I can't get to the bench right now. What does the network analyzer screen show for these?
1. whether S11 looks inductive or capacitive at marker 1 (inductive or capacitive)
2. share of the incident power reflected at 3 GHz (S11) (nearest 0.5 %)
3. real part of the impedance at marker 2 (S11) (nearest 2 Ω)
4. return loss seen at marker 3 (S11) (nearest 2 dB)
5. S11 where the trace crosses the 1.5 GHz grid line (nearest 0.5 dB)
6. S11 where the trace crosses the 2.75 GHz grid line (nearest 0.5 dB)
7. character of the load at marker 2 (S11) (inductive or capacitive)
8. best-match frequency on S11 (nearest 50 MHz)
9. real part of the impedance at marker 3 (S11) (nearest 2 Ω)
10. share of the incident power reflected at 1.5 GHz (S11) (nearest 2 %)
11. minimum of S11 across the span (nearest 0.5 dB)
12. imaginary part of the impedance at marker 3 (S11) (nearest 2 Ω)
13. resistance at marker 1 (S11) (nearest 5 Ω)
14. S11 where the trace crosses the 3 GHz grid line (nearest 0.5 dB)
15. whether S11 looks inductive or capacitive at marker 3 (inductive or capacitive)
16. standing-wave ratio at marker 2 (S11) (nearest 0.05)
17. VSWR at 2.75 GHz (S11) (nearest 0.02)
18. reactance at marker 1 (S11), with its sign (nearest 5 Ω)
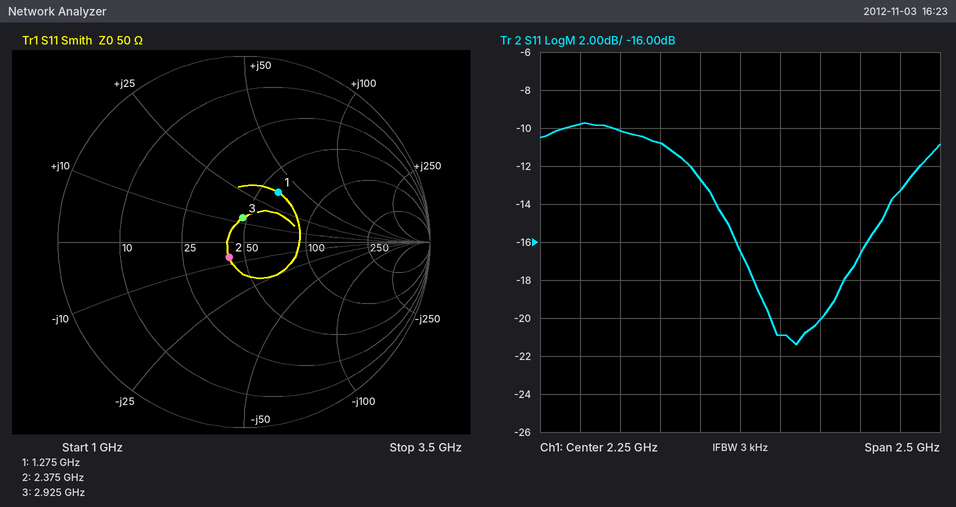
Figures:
inductive
2.0 %
42 Ω
18 dB
-10.0 dB
-20.0 dB
capacitive
2.60 GHz
48 Ω
10 %
-21.5 dB
+12 Ω
60 Ω
-16.5 dB
inductive
1.25
1.22
+35 Ω
